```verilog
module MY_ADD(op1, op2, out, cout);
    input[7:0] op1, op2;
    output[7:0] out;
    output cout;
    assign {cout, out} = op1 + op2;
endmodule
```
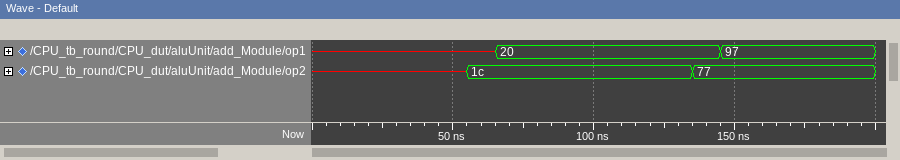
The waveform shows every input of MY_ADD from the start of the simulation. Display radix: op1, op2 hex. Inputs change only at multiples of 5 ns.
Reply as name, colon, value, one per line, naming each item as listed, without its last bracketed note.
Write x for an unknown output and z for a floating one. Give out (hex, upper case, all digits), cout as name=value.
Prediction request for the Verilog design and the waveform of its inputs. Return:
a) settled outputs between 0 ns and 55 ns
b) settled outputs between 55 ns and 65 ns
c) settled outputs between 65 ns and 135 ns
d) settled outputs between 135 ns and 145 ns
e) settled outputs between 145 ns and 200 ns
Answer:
settled outputs between 0 ns and 55 ns: out=x, cout=x
settled outputs between 55 ns and 65 ns: out=x, cout=x
settled outputs between 65 ns and 135 ns: out=3C, cout=0
settled outputs between 135 ns and 145 ns: out=97, cout=0
settled outputs between 145 ns and 200 ns: out=0E, cout=1
